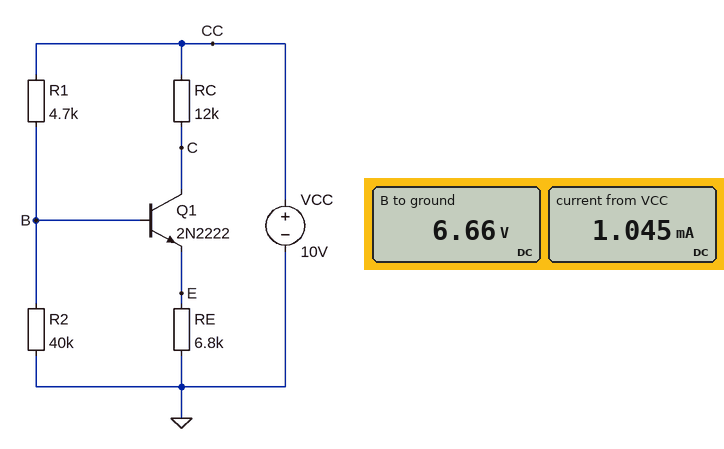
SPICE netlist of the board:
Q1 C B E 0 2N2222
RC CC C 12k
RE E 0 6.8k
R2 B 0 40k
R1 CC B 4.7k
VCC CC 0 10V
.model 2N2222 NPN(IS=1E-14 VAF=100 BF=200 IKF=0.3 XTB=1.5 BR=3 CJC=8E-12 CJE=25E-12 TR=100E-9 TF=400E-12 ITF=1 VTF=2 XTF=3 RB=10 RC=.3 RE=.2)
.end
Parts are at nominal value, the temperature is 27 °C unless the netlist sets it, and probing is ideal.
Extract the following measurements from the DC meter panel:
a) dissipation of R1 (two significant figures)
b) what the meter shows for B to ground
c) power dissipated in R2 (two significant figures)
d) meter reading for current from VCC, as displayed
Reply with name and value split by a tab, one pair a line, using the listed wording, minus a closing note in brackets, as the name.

dissipation of R1	2.4 mW
what the meter shows for B to ground	6.66 V
power dissipated in R2	1.1 mW
meter reading for current from VCC, as displayed	1.045 mA
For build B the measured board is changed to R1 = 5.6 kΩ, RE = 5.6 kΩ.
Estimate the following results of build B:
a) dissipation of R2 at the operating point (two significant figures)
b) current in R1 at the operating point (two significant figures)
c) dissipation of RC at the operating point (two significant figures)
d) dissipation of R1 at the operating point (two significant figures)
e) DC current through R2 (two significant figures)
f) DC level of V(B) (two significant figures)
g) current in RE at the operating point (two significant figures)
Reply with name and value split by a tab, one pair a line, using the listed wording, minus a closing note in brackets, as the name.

dissipation of R2 at the operating point	900 µW
current in R1 at the operating point	710 µA
dissipation of RC at the operating point	1.8 mW
dissipation of R1 at the operating point	2.8 mW
DC current through R2	150 µA
DC level of V(B)	6.0 V
current in RE at the operating point	950 µA
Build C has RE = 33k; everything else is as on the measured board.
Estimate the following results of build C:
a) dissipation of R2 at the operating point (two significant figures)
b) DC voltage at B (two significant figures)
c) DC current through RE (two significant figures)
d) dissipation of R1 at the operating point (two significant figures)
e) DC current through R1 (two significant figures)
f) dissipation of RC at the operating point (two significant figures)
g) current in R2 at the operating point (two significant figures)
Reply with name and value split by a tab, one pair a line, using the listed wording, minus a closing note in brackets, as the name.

dissipation of R2 at the operating point	1.9 mW
DC voltage at B	8.6 V
DC current through RE	240 µA
dissipation of R1 at the operating point	400 µW
DC current through R1	290 µA
dissipation of RC at the operating point	330 µW
current in R2 at the operating point	220 µA
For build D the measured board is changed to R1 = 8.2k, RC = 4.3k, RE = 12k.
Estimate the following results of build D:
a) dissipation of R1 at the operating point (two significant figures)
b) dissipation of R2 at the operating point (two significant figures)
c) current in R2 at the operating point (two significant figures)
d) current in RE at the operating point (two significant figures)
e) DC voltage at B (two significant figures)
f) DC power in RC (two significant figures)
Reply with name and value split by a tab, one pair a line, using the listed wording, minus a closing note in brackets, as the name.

dissipation of R1 at the operating point	450 µW
dissipation of R2 at the operating point	1.6 mW
current in R2 at the operating point	200 µA
current in RE at the operating point	620 µA
DC voltage at B	8.1 V
DC power in RC	1.5 mW
